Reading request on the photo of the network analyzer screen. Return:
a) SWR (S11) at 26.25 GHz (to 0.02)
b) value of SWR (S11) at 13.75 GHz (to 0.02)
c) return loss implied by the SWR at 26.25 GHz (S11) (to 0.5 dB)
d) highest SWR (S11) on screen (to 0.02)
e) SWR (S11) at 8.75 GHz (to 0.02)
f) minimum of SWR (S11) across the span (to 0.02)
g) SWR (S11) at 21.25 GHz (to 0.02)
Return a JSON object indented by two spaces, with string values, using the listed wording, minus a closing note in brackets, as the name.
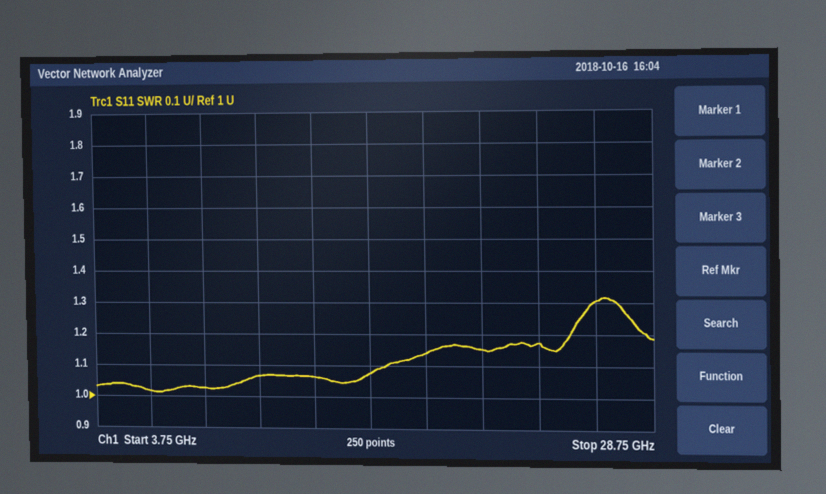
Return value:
{
  "SWR (S11) at 26.25 GHz": "1.30",
  "value of SWR (S11) at 13.75 GHz": "1.06",
  "return loss implied by the SWR at 26.25 GHz (S11)": "17.5 dB",
  "highest SWR (S11) on screen": "1.32",
  "SWR (S11) at 8.75 GHz": "1.02",
  "minimum of SWR (S11) across the span": "1.02",
  "SWR (S11) at 21.25 GHz": "1.16"
}
